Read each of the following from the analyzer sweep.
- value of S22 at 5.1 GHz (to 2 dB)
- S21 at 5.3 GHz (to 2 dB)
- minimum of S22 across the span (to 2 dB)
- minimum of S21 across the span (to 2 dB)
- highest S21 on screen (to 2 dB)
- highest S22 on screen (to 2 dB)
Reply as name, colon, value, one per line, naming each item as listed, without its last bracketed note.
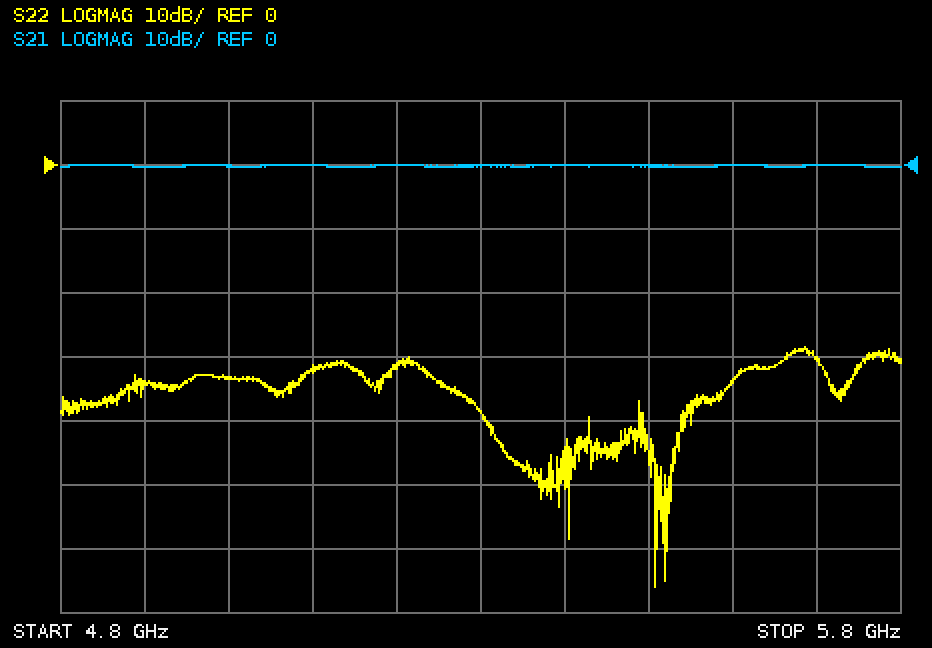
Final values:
value of S22 at 5.1 GHz: -32 dB
S21 at 5.3 GHz: 0 dB
minimum of S22 across the span: -66 dB
minimum of S21 across the span: 0 dB
highest S21 on screen: 0 dB
highest S22 on screen: -28 dB
